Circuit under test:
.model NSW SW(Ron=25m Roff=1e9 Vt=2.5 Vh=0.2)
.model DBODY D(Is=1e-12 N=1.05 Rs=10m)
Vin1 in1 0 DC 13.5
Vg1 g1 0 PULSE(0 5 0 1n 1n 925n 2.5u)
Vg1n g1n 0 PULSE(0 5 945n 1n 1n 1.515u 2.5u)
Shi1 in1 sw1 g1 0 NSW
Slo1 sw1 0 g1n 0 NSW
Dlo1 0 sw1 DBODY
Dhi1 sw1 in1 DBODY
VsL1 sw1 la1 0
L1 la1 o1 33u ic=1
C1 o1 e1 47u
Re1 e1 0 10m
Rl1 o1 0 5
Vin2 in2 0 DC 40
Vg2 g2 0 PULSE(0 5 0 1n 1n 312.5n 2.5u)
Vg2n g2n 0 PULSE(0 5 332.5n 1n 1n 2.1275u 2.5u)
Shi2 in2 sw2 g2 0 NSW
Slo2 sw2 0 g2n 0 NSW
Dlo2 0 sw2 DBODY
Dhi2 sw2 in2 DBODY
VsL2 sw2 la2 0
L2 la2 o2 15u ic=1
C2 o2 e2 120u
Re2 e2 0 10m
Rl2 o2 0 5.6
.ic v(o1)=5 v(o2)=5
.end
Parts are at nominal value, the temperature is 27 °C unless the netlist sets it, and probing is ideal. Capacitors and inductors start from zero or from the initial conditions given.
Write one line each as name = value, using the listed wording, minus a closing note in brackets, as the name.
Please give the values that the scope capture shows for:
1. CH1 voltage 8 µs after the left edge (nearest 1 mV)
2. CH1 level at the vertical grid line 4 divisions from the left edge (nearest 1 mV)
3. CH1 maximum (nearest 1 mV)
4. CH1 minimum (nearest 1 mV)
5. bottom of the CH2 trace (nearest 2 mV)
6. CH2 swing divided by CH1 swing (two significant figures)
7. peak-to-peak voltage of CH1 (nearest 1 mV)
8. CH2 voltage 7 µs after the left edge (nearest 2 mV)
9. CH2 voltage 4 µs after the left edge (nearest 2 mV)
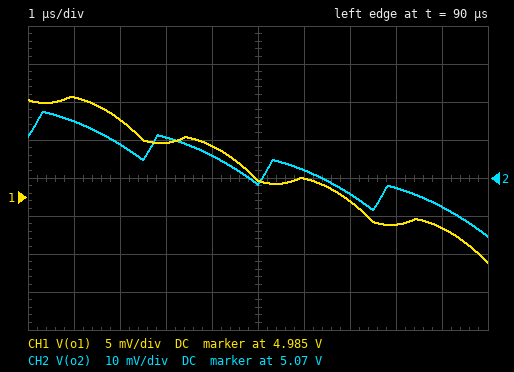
CH1 voltage 8 µs after the left edge = 4.981 V
CH1 level at the vertical grid line 4 divisions from the left edge = 4.992 V
CH1 maximum = 4.998 V
CH1 minimum = 4.976 V
bottom of the CH2 trace = 5.054 V
CH2 swing divided by CH1 swing = 1.5
peak-to-peak voltage of CH1 = 22 mV
CH2 voltage 7 µs after the left edge = 5.066 V
CH2 voltage 4 µs after the left edge = 5.076 V
